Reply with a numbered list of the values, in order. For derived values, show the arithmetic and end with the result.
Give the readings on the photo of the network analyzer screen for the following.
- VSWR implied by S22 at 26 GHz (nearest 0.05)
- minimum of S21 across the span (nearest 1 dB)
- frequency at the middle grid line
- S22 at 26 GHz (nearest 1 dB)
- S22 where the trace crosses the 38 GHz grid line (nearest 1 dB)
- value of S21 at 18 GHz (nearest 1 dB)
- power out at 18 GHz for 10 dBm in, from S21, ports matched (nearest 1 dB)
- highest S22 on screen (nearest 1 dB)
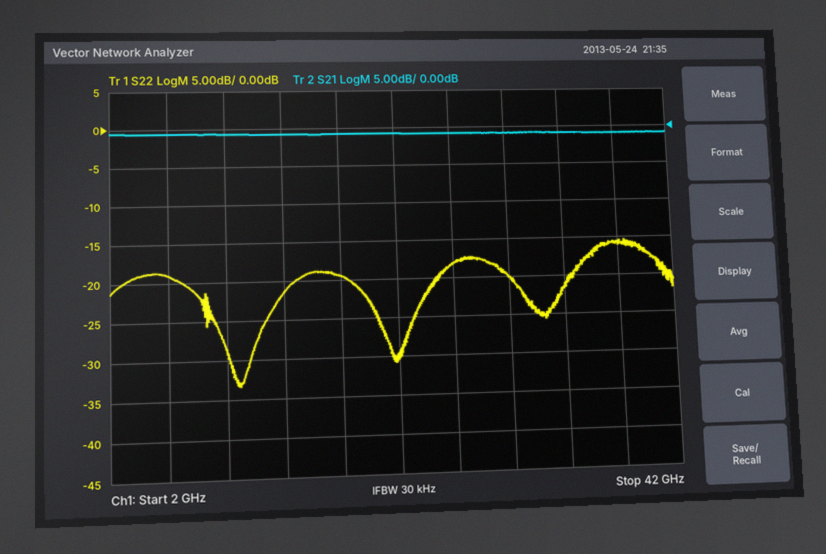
1. |Γ| = 10^(-18/20) = 0.1259; VSWR = (1 + 0.1259)/(1 − 0.1259) ≈ 1.29, so 1.30 to the nearest 0.05
2. -1 dB
3. 22 GHz
4. -18 dB
5. -16 dB
6. -1 dB
7. 10 dBm + (-1 dB) = 9 dBm
8. -15 dB
